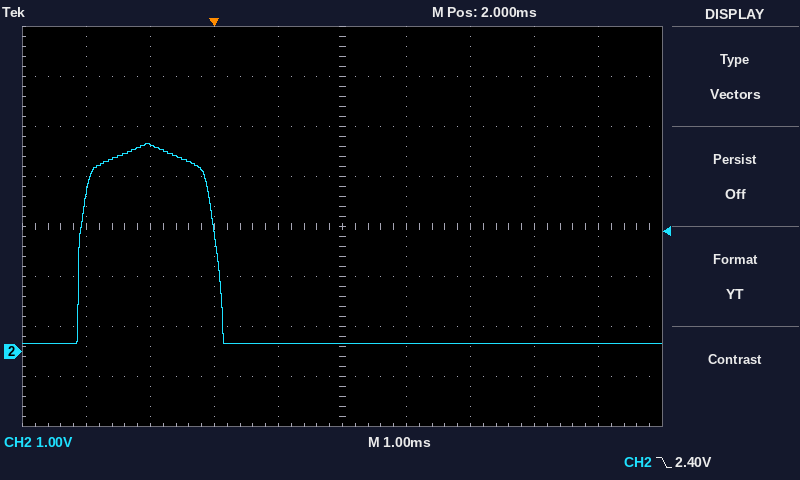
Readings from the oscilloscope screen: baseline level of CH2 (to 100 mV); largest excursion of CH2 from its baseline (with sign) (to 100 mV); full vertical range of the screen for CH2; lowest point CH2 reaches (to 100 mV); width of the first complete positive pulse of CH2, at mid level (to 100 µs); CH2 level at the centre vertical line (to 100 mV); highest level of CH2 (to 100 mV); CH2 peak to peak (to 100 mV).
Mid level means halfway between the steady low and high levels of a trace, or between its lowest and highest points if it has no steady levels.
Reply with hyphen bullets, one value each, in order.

- 200 mV
- +4.0 V
- 8 V
- 200 mV
- 2.1 ms
- 200 mV
- 4.2 V
- 4.0 V
